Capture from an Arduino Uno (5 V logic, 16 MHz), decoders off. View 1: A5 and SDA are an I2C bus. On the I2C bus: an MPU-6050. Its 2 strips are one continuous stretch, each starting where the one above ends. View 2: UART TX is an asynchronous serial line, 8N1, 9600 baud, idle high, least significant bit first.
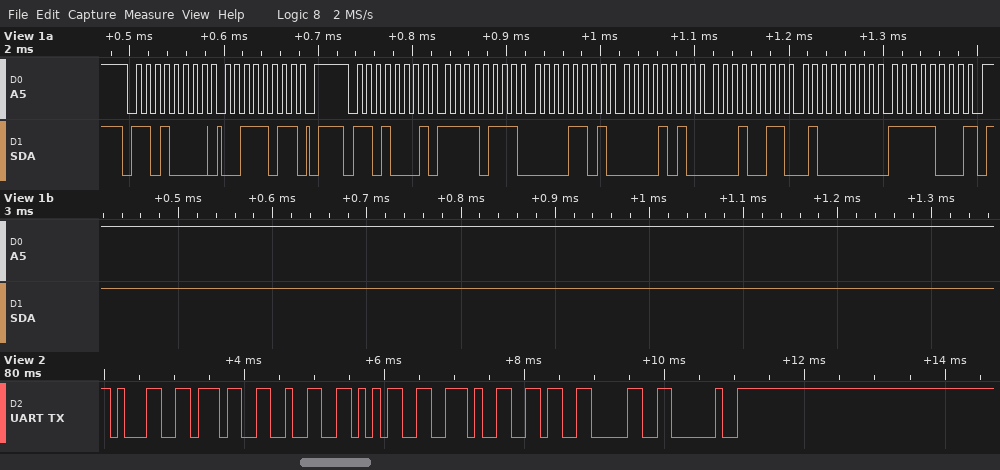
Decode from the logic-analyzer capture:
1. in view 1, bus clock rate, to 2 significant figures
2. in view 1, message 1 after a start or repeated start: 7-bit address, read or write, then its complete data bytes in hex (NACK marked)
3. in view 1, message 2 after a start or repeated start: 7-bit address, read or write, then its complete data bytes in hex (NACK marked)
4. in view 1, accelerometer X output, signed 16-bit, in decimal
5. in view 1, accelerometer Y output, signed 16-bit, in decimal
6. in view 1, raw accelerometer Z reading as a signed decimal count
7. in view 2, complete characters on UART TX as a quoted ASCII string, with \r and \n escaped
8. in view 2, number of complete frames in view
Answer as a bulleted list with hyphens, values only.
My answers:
- 100 kHz
- 0x68 write: 3B
- 0x68 read: F7 0D 0A 13 40 F8 NACK
- -2291
- 2579
- 16632
- "1725.60 "
- 8
